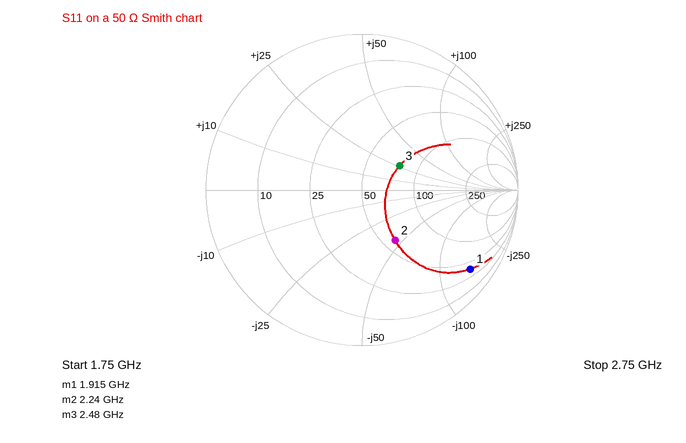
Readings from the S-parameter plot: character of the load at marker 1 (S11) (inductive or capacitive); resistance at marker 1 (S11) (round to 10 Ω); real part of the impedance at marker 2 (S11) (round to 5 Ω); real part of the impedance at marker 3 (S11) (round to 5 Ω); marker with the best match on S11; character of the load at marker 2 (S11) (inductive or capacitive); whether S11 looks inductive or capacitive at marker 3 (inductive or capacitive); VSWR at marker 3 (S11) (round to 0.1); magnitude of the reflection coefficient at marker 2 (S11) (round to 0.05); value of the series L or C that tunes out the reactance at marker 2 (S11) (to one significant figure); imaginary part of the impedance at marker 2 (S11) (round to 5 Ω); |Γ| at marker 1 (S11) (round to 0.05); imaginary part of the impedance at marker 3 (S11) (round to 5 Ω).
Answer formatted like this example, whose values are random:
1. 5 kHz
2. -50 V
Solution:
1. capacitive
2. 40 Ω
3. 60 Ω
4. 75 Ω
5. marker 3
6. capacitive
7. inductive
8. 1.8
9. 0.40
10. 3 nH
11. -45 Ω
12. 0.85
13. +25 Ω
